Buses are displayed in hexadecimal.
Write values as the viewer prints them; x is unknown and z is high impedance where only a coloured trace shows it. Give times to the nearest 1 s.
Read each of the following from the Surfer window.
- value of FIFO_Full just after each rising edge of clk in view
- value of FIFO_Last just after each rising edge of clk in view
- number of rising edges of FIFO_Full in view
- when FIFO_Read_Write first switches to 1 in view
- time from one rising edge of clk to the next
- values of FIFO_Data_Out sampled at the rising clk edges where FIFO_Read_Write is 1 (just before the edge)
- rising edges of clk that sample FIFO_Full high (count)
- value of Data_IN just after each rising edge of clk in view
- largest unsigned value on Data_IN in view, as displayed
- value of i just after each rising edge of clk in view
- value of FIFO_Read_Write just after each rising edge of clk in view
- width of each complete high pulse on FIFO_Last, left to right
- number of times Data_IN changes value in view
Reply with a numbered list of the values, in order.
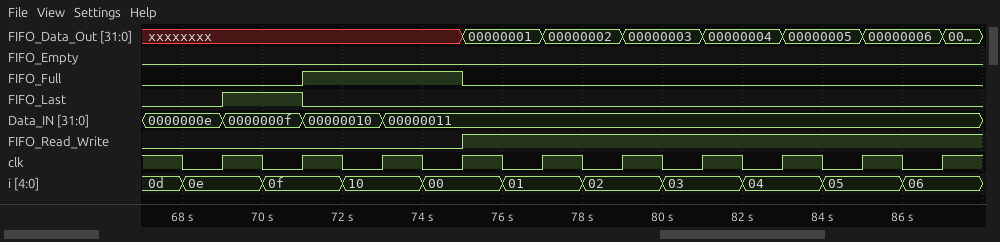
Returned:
1. 0 1 1 0 0 0 0 0 0 0
2. 1 0 0 0 0 0 0 0 0 0
3. 1
4. 75 s
5. 2 s
6. 00000001, 00000002, 00000003, 00000004, 00000005, 00000006
7. 2
8. 0000000f, 00000010, 00000011, 00000011, 00000011, 00000011, 00000011, 00000011, 00000011, 00000011
9. 00000011
10. 0e, 0f, 10, 00, 01, 02, 03, 04, 05, 06
11. 0 0 0 1 1 1 1 1 1 1
12. 2 s
13. 3
